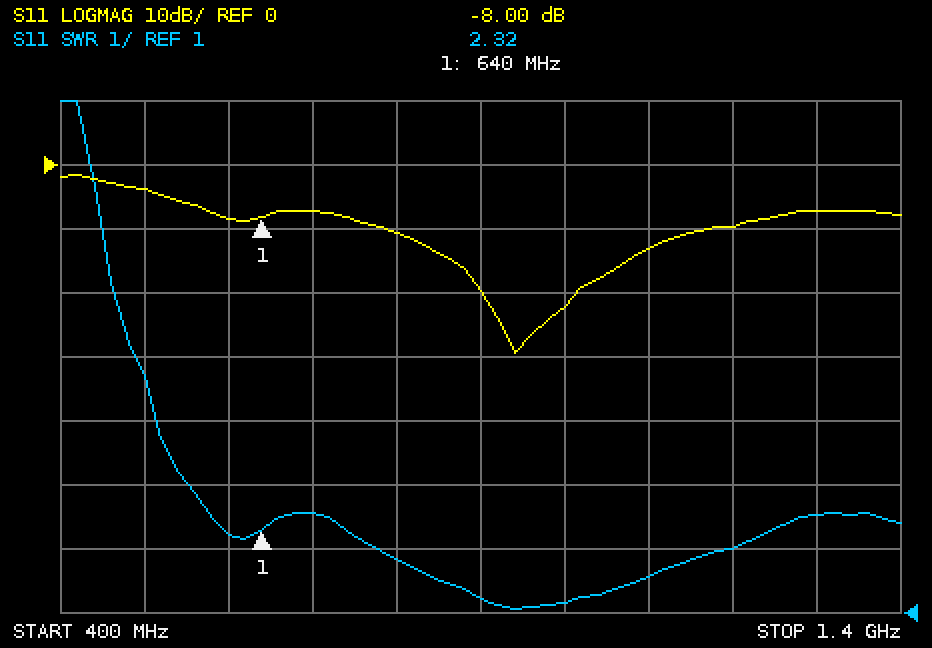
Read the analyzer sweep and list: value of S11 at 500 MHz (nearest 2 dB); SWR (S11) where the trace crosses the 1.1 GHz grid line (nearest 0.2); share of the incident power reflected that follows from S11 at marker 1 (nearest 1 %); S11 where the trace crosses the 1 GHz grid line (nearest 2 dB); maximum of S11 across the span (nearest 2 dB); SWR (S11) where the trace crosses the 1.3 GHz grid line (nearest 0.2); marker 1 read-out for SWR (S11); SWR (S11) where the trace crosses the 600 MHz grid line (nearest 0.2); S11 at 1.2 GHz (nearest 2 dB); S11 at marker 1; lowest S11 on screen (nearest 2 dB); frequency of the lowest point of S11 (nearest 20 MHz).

-4 dB
1.6
16 %
-22 dB
-2 dB
2.6
2.32
2.2
-10 dB
-8.00 dB
-30 dB
940 MHz
